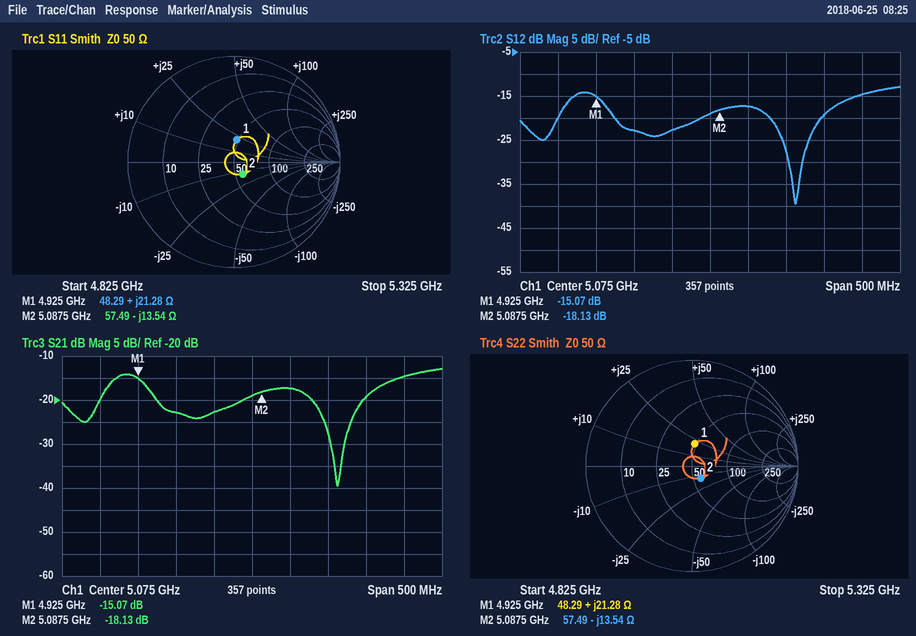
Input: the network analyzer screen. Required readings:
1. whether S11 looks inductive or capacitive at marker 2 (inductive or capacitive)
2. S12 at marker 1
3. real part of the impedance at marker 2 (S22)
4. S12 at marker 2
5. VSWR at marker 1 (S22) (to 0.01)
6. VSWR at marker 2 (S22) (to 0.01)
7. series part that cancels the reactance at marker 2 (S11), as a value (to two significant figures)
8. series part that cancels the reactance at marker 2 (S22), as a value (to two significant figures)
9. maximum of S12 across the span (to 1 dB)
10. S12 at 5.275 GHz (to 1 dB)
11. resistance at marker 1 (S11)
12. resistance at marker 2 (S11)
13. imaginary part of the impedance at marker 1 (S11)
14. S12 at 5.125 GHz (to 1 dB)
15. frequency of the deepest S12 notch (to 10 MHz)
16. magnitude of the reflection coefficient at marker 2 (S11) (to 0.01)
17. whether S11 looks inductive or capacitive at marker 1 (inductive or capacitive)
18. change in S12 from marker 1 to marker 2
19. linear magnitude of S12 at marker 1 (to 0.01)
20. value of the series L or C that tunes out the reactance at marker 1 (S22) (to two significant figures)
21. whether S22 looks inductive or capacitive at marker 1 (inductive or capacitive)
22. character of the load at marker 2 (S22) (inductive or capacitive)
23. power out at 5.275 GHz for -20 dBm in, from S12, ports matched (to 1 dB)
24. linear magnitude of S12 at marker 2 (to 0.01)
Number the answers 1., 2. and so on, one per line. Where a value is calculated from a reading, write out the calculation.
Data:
1. capacitive
2. -15.07 dB
3. 57.49 Ω
4. -18.13 dB
5. 1.54
6. 1.33
7. L = 13.54 Ω/(2π × 5.0875 GHz) ≈ 424 pH, so 420 pH to two significant figures
8. L = 13.54 Ω/(2π × 5.0875 GHz) ≈ 424 pH, so 420 pH to two significant figures
9. -13 dB
10. -15 dB
11. 48.29 Ω
12. 57.49 Ω
13. +21.28 Ω
14. -17 dB
15. 5.19 GHz
16. 0.14
17. inductive
18. -18.13 − (-15.07) = -3.06 dB
19. 10^(-15.07/20) ≈ 0.18
20. C = 1/(2π × 4.925 GHz × 21.28 Ω) ≈ 1.5 pF
21. inductive
22. capacitive
23. -20 dBm + (-15 dB) = -35 dBm
24. 10^(-18.13/20) ≈ 0.12
